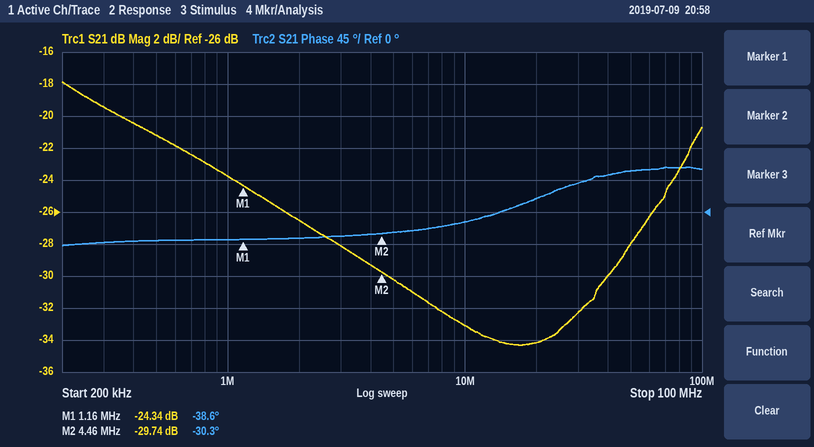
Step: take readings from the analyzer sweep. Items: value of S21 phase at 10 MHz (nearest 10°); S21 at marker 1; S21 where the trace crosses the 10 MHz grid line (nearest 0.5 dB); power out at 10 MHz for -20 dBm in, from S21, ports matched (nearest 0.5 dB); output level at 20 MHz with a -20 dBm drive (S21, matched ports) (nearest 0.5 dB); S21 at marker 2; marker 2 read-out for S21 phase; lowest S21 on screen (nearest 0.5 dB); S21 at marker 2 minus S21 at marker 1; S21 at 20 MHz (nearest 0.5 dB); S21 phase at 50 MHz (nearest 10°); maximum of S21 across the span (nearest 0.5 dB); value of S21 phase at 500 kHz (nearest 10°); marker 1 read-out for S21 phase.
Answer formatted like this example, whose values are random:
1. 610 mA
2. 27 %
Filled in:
1. -10°
2. -24.34 dB
3. -33.0 dB
4. -53.0 dBm
5. -54.0 dBm
6. -29.74 dB
7. -30.3°
8. -34.5 dB
9. -5.40 dB
10. -34.0 dB
11. 60°
12. -18.0 dB
13. -40°
14. -38.6°
